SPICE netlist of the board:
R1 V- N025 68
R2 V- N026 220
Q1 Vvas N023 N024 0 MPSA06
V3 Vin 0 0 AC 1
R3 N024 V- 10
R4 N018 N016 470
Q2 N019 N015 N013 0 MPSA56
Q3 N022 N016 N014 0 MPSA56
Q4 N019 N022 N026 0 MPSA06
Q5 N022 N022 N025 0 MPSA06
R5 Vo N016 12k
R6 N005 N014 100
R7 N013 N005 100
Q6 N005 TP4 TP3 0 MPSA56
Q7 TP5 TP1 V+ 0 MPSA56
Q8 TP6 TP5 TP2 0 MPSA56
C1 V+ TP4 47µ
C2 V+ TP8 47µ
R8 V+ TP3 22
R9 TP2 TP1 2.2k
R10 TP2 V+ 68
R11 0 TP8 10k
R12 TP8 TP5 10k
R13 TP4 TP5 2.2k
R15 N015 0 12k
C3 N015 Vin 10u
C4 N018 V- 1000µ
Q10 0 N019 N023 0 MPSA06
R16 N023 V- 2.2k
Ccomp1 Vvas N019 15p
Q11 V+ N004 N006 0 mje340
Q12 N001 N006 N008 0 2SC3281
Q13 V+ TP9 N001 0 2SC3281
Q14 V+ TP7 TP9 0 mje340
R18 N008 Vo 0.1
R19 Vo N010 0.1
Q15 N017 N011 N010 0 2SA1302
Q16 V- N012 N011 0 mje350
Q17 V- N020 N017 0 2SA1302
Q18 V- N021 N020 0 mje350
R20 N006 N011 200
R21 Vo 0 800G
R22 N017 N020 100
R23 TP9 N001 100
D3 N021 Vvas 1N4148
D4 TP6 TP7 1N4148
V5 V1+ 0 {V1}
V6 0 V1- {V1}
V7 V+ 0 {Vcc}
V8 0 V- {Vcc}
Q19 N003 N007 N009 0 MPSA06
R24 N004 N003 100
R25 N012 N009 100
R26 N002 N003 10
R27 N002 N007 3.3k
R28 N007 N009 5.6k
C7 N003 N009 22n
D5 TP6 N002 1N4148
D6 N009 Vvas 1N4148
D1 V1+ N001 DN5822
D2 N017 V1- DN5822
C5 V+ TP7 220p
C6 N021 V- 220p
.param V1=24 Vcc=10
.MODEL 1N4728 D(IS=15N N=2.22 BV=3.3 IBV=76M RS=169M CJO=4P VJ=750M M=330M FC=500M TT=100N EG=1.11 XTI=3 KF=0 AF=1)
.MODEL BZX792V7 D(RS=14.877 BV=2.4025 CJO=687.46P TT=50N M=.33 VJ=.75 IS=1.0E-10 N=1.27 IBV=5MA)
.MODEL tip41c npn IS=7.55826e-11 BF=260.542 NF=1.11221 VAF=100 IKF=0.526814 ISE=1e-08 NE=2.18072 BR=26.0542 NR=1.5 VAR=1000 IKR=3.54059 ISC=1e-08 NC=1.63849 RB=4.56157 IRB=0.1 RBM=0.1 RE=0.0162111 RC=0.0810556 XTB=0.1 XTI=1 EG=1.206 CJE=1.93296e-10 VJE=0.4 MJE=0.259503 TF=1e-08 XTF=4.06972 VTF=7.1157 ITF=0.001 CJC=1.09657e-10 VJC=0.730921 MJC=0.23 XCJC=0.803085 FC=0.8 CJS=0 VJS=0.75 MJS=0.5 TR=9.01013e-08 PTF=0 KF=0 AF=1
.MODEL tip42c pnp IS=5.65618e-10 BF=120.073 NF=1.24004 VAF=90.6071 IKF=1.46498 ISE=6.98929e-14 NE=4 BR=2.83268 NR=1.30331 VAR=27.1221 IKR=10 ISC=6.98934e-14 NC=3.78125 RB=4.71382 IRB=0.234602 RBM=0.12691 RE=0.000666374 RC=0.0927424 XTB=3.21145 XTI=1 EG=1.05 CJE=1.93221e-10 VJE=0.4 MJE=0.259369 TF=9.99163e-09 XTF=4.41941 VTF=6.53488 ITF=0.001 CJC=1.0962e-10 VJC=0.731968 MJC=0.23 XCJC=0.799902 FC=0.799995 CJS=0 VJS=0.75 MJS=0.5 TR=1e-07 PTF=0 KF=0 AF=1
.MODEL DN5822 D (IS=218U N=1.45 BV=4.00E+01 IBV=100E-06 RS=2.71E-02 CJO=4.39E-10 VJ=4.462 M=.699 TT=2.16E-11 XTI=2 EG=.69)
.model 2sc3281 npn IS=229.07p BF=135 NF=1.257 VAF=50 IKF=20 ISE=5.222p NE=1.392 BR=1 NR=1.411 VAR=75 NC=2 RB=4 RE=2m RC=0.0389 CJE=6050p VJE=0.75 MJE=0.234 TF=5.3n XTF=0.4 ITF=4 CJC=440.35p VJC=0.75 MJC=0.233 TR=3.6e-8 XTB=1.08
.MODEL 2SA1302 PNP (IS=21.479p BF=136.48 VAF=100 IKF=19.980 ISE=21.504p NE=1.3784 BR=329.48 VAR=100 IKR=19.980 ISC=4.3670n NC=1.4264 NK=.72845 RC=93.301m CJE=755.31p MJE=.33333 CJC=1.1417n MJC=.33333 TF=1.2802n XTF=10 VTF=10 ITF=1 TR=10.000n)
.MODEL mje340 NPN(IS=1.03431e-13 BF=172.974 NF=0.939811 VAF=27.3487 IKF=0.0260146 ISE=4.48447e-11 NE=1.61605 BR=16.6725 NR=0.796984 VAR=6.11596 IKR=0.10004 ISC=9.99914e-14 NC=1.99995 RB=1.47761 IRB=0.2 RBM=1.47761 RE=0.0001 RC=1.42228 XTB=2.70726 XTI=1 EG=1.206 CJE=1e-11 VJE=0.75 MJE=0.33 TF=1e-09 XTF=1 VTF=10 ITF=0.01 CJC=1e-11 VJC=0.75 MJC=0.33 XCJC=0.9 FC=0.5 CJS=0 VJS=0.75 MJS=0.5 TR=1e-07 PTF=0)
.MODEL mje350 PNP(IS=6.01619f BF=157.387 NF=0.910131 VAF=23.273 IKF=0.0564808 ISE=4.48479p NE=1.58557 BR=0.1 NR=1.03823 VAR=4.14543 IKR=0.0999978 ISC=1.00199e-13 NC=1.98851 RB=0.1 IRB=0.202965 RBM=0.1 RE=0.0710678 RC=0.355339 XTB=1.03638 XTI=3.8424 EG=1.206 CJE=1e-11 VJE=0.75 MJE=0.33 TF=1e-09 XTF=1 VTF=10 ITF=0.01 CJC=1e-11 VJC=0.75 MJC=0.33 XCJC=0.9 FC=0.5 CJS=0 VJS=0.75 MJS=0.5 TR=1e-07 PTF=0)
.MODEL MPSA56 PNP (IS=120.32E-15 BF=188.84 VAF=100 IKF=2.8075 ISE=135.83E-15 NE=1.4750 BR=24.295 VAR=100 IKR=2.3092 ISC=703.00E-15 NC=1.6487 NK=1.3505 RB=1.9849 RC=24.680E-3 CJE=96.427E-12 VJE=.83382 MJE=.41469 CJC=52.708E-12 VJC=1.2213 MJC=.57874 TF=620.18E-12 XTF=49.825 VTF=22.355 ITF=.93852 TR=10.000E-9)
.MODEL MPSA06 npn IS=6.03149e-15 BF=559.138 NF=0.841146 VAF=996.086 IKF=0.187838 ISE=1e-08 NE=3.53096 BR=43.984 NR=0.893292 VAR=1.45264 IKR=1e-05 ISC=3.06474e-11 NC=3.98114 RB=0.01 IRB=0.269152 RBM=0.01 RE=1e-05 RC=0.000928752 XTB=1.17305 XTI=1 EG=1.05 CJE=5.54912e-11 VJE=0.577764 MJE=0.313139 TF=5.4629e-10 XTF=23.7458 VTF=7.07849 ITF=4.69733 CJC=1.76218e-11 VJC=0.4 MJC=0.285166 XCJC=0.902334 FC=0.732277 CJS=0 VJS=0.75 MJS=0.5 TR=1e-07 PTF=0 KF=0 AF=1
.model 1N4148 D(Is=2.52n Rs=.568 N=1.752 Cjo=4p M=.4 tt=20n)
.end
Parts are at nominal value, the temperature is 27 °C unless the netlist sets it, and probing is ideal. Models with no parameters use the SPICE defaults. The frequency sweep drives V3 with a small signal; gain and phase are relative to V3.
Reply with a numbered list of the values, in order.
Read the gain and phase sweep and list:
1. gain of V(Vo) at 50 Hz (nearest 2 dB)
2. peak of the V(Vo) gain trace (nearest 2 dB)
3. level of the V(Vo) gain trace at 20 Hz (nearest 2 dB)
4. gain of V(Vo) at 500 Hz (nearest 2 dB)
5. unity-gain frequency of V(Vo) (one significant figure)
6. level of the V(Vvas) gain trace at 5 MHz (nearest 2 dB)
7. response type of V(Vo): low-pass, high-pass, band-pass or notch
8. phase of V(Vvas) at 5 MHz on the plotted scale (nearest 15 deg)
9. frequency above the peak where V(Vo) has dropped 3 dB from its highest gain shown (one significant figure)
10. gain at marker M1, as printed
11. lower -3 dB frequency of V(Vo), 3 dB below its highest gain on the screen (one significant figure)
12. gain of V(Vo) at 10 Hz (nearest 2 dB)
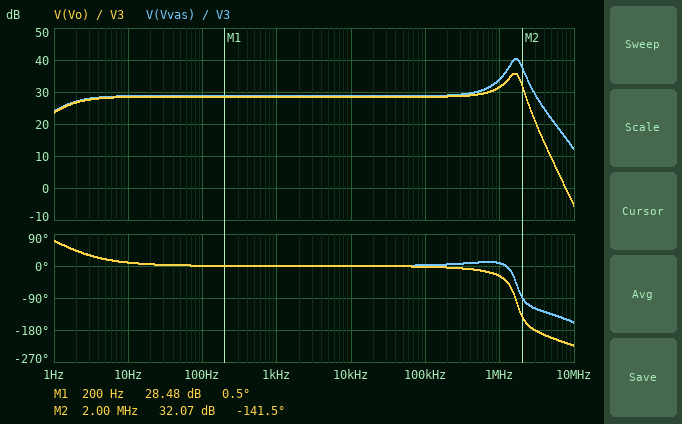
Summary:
1. 28 dB
2. 36 dB
3. 28 dB
4. 28 dB
5. 8 MHz
6. 22 dB
7. band-pass
8. -135 deg
9. 2 MHz
10. 28.48 dB
11. 1 MHz
12. 28 dB
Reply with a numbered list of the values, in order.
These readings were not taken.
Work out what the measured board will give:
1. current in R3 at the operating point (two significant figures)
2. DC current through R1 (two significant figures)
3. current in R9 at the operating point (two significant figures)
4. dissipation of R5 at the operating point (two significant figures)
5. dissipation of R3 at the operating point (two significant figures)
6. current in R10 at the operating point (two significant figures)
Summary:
1. 8.3 mA
2. 12 mA
3. 2.0 µA
4. 50 µW
5. 690 µW
6. 8.3 mA
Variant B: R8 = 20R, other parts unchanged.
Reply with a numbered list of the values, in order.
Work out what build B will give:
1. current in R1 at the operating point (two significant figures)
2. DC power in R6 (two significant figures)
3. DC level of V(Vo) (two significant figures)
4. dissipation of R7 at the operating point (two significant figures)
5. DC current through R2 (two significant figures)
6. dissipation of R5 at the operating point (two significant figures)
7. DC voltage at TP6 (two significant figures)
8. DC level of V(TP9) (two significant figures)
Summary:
1. 13 mA
2. 17 mW
3. -1.5 V
4. 1.7 mW
5. 4.1 mA
6. 56 µW
7. -610 mV
8. 11 V
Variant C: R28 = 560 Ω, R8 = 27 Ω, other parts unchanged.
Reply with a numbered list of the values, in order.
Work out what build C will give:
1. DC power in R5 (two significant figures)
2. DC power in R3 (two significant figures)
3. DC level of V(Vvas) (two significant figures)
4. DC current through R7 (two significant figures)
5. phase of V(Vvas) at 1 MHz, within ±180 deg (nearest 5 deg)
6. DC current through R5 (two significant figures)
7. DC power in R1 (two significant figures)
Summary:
1. 39 µW
2. 650 µW
3. -3.9 V
4. 3.4 mA
5. -20 deg
6. 57 µA
7. 7.8 mW
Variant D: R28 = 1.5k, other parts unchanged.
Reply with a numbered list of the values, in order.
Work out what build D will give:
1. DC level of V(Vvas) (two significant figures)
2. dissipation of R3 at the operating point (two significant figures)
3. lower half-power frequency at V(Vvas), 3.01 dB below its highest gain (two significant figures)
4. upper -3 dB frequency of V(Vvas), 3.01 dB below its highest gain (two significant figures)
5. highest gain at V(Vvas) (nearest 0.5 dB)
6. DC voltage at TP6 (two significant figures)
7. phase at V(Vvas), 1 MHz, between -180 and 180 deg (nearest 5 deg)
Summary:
1. -3.1 V
2. 680 µW
3. 1.4 Hz
4. 4.5 MHz
5. 28.5 dB
6. 350 mV
7. -20 deg
